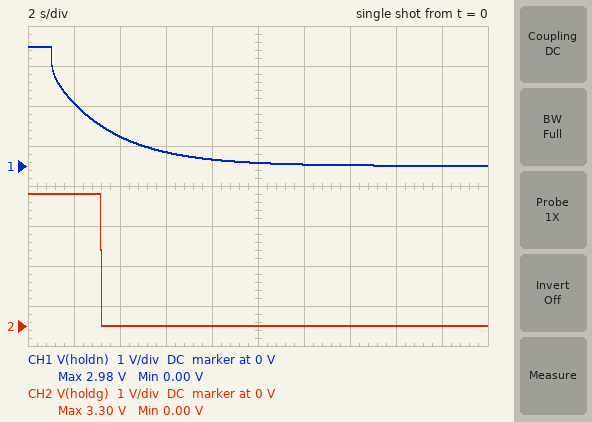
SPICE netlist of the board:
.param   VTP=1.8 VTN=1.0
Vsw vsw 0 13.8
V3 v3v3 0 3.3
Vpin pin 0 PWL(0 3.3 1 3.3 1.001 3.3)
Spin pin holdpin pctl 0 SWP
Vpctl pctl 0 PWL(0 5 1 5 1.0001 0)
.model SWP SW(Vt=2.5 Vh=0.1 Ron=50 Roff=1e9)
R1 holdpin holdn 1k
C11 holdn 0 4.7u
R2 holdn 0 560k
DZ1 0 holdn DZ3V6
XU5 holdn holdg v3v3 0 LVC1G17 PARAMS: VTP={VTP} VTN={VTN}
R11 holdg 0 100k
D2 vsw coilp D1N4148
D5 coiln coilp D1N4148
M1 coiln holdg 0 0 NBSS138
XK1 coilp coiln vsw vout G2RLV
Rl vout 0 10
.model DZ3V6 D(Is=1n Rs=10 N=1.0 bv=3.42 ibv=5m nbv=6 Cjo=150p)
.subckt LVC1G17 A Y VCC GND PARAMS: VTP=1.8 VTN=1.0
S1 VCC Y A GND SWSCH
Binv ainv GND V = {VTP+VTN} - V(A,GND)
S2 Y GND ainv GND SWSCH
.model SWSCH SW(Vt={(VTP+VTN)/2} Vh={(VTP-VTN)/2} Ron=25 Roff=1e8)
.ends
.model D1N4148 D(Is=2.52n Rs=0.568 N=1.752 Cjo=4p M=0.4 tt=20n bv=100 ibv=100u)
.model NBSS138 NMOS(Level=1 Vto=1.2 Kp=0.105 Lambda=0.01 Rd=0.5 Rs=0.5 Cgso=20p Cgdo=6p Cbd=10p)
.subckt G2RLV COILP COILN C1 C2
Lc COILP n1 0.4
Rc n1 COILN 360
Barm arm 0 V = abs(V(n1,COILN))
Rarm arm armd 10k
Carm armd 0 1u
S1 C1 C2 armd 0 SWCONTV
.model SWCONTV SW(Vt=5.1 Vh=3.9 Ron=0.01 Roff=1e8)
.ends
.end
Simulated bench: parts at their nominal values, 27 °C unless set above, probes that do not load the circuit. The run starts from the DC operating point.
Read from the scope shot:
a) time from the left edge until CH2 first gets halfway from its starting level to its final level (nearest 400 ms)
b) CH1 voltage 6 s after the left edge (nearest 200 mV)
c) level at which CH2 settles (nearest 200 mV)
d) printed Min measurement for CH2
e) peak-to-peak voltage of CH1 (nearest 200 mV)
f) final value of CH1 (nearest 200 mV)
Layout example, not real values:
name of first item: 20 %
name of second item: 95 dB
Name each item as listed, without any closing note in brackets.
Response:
time from the left edge until CH2 first gets halfway from its starting level to its final level: 3.2 s
CH1 voltage 6 s after the left edge: 400 mV
level at which CH2 settles: 0 V
printed Min measurement for CH2: 0.00 V
peak-to-peak voltage of CH1: 3.0 V
final value of CH1: 0 V
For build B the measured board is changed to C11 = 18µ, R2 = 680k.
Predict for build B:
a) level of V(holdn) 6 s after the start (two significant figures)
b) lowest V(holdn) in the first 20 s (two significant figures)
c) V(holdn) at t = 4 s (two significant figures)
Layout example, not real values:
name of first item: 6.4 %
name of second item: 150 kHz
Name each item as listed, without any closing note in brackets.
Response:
level of V(holdn) 6 s after the start: 1.5 V
lowest V(holdn) in the first 20 s: 480 mV
V(holdn) at t = 4 s: 1.8 V
